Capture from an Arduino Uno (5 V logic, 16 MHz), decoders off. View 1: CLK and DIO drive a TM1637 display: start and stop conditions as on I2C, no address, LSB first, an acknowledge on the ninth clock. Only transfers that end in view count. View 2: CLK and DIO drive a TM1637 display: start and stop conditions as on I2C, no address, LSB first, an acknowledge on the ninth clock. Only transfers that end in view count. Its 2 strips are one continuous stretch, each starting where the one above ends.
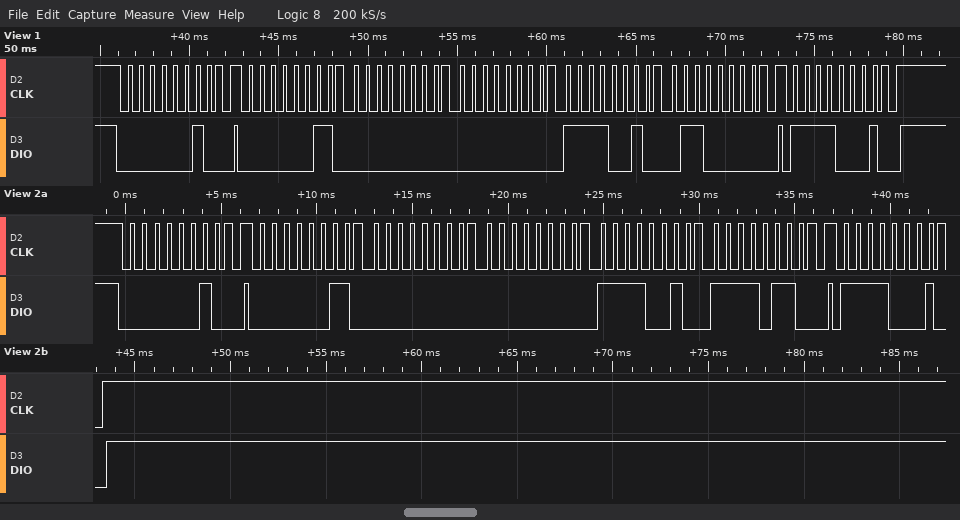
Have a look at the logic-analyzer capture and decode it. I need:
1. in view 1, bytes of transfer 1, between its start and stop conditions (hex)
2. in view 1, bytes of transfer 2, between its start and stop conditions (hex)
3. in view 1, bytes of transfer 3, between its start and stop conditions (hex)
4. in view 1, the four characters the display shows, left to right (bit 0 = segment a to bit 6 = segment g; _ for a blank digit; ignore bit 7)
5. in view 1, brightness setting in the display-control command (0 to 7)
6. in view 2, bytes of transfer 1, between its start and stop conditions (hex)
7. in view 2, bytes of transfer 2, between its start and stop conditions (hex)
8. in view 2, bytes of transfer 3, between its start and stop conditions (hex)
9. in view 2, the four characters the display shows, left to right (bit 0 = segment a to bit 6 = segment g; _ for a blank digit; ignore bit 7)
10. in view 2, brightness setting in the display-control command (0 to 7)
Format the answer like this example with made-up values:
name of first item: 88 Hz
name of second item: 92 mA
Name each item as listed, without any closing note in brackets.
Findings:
in view 1, bytes of transfer 1, between its start and stop conditions: 40
in view 1, bytes of transfer 2, between its start and stop conditions: C0 00 00 4F 06
in view 1, bytes of transfer 3, between its start and stop conditions: 8F
in view 1, the four characters the display shows, left to right: __31
in view 1, brightness setting in the display-control command: 7
in view 2, bytes of transfer 1, between its start and stop conditions: 40
in view 2, bytes of transfer 2, between its start and stop conditions: C0 00 00 4F 6F
in view 2, bytes of transfer 3, between its start and stop conditions: 8F
in view 2, the four characters the display shows, left to right: __39
in view 2, brightness setting in the display-control command: 7
